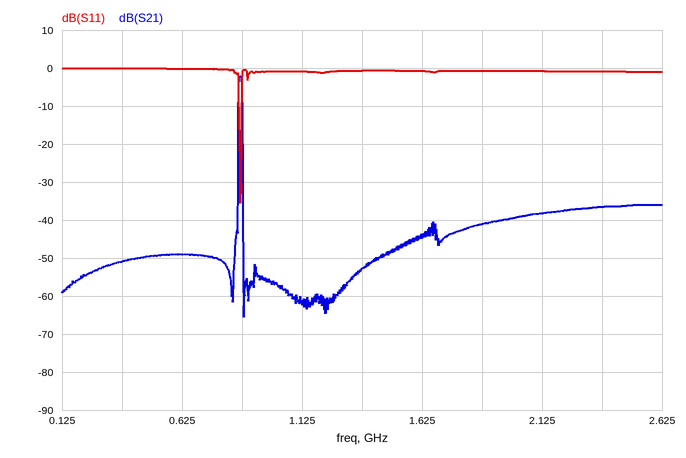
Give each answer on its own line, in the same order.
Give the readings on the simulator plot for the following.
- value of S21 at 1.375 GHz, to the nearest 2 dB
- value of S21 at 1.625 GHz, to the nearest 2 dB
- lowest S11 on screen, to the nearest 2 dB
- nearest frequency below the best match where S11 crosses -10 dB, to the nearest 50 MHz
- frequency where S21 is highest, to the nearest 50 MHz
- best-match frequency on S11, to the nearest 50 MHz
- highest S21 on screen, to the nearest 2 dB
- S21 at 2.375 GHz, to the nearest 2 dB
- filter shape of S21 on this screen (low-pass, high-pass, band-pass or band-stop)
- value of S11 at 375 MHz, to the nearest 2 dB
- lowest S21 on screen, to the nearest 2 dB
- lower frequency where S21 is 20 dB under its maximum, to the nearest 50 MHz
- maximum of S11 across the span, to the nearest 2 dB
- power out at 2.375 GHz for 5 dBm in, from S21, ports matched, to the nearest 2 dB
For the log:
-52 dB
-44 dB
-36 dB
850 MHz
850 MHz
850 MHz
-2 dB
-36 dB
band-pass
0 dB
-66 dB
850 MHz
0 dB
-32 dBm
